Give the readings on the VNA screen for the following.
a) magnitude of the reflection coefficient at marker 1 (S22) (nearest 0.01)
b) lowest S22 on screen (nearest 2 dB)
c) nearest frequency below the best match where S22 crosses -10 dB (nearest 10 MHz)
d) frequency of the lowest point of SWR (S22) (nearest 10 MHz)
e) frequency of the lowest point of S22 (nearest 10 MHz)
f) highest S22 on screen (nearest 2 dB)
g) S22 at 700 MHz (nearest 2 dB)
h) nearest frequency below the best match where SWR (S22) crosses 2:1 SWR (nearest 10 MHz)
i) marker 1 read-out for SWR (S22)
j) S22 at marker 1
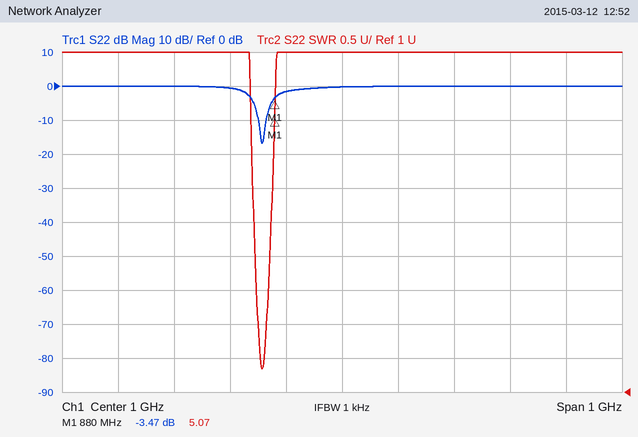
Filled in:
0.67
-16 dB
850 MHz
860 MHz
860 MHz
0 dB
0 dB
850 MHz
5.07
-3.47 dB
